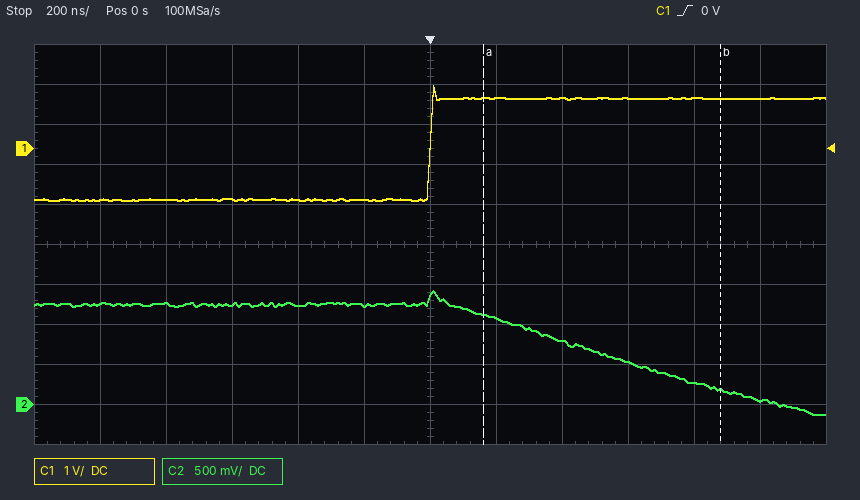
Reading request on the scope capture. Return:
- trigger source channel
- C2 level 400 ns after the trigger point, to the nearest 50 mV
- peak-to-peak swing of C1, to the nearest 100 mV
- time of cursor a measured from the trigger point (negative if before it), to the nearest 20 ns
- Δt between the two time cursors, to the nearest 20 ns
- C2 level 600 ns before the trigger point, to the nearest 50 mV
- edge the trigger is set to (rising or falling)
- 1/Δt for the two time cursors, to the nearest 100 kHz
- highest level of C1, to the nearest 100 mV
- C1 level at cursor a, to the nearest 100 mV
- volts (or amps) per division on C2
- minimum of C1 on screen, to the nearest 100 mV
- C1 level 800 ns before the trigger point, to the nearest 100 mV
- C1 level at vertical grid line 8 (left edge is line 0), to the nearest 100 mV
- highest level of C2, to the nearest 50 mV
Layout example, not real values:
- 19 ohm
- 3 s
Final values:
- C1
- 800 mV
- 2.9 V
- +160 ns
- 720 ns
- 1.25 V
- rising
- 1.4 MHz
- 1.6 V
- 1.3 V
- 500 mV
- -1.3 V
- -1.3 V
- 1.3 V
- 1.40 V
